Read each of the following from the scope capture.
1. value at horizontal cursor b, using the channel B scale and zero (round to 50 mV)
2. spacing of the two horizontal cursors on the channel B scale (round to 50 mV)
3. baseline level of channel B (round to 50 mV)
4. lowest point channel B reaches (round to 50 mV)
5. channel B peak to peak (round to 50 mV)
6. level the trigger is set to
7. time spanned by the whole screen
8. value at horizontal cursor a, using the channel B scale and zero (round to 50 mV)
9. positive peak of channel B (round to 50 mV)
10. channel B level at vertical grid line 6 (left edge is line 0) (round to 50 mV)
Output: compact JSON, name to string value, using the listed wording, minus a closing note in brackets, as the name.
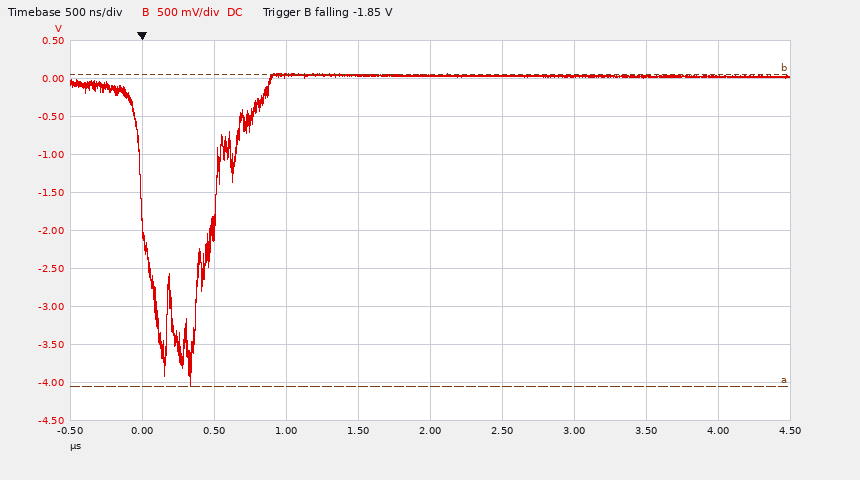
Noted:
{"value at horizontal cursor b, using the channel B scale and zero": "50 mV", "spacing of the two horizontal cursors on the channel B scale": "4.10 V", "baseline level of channel B": "50 mV", "lowest point channel B reaches": "-4.05 V", "channel B peak to peak": "4.10 V", "level the trigger is set to": "-1.85 V", "time spanned by the whole screen": "5 µs", "value at horizontal cursor a, using the channel B scale and zero": "-4.05 V", "positive peak of channel B": "50 mV", "channel B level at vertical grid line 6 (left edge is line 0)": "50 mV"}
